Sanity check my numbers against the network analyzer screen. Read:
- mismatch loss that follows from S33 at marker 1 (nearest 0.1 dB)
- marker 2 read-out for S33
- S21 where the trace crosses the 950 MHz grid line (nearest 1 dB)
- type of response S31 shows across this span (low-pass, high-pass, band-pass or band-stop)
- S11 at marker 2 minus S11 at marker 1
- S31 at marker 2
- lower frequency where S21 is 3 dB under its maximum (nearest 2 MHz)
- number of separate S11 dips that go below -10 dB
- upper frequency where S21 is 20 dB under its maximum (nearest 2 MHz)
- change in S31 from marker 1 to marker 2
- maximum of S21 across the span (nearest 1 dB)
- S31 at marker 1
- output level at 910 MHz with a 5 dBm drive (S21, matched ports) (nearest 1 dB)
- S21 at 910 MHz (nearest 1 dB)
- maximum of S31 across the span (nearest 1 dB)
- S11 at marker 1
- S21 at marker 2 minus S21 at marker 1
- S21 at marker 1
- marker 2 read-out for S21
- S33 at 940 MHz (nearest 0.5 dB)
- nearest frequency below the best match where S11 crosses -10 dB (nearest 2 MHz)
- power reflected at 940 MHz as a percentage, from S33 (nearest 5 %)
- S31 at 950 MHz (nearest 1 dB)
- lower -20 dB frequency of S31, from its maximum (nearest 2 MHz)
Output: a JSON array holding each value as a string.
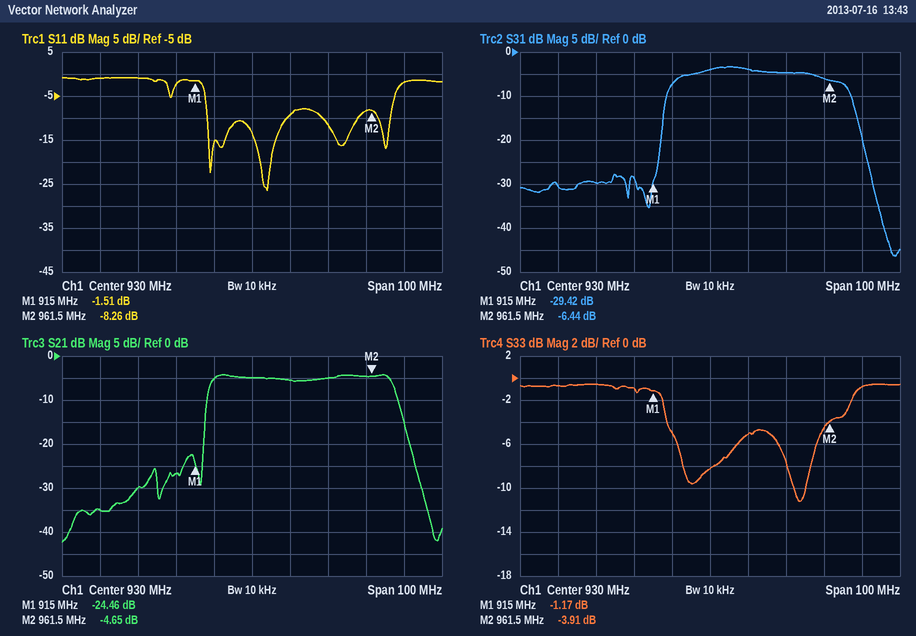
["6.3 dB", "-3.91 dB", "-5 dB", "band-pass", "-6.75 dB", "-6.44 dB", "918 MHz", "4", "972 MHz", "22.98 dB", "-4 dB", "-29.42 dB", "-22 dBm", "-27 dB", "-3 dB", "-1.51 dB", "19.81 dB", "-24.46 dB", "-4.65 dB", "-5.0 dB", "918 MHz", "30 %", "-5 dB", "916 MHz"]
